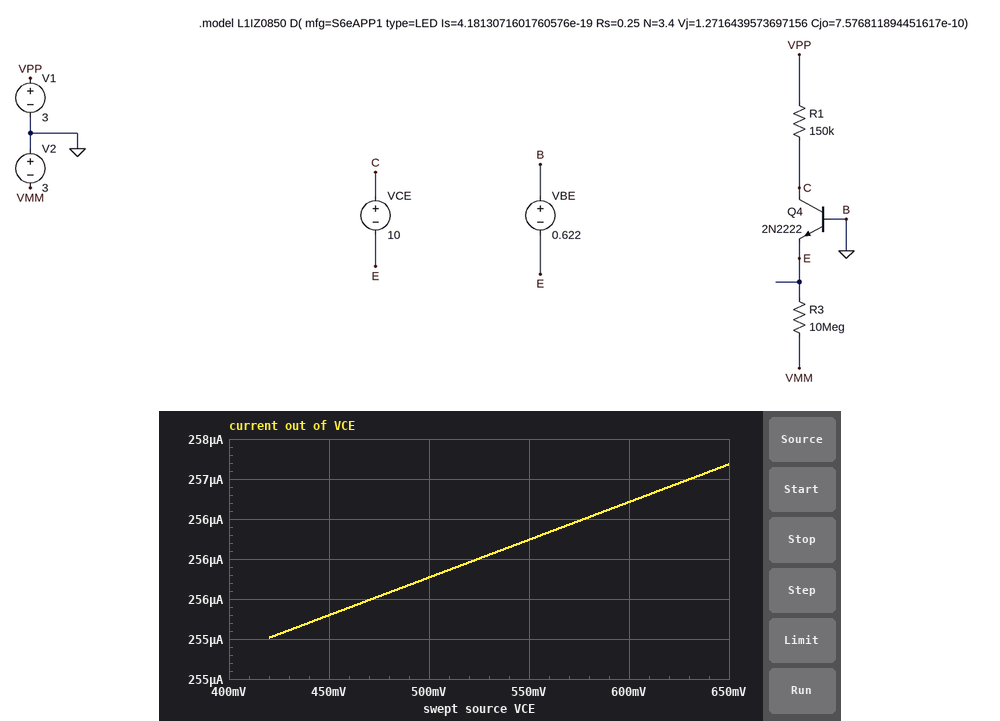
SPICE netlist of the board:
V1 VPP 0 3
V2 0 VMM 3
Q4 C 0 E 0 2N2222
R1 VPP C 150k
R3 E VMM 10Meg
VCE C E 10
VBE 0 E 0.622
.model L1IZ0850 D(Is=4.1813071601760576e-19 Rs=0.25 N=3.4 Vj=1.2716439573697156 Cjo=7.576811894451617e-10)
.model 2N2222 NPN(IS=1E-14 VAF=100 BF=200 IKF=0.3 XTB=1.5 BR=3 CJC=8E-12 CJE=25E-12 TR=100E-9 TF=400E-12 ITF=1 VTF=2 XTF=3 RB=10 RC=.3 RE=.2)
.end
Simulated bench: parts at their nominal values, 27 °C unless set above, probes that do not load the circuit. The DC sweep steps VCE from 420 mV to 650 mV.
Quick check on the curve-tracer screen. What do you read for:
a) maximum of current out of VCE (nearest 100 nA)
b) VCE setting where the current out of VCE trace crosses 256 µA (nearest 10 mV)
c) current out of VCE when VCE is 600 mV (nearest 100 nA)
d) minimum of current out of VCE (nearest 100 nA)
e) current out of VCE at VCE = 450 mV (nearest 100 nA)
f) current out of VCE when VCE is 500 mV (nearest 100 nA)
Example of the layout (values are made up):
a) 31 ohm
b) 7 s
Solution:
a) 257.2 µA
b) 580 mV
c) 256.7 µA
d) 255.0 µA
e) 255.3 µA
f) 255.8 µA
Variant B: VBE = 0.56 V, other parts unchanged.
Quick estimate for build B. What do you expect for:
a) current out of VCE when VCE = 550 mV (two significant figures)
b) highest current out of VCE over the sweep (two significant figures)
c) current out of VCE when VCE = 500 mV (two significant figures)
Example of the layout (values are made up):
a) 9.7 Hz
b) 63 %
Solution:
a) 5.2 µA
b) 5.9 µA
c) 4.9 µA
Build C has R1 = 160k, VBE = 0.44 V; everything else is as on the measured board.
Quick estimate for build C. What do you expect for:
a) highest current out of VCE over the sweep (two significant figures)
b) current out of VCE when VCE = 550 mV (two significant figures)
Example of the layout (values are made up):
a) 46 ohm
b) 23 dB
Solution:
a) -17 µA
b) -18 µA
